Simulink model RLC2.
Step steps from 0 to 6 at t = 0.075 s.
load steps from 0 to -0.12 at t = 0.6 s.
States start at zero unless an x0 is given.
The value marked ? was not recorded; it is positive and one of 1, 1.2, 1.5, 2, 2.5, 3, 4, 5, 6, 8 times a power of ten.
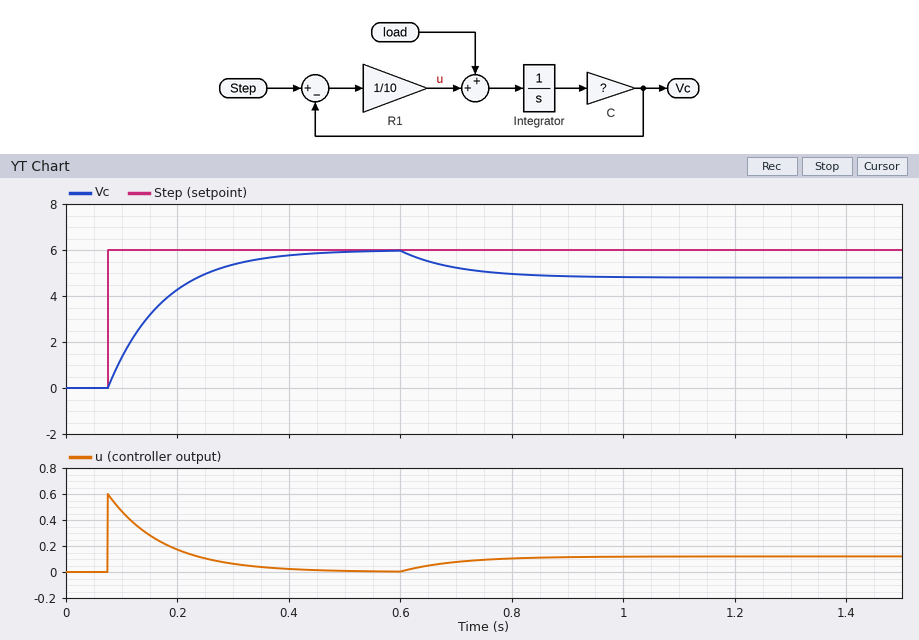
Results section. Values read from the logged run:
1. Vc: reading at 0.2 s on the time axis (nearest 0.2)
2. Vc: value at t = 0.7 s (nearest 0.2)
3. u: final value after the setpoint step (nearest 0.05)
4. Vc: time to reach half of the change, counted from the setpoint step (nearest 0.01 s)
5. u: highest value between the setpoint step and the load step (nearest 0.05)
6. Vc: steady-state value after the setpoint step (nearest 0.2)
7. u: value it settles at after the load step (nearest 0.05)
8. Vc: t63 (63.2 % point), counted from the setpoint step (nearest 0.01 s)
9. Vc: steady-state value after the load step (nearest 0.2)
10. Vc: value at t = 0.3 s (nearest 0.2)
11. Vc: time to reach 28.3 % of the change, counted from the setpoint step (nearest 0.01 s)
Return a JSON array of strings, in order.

["4.2", "5.2", "0.00", "0.07 s", "0.60", "6.0", "0.10", "0.10 s", "4.8", "5.4", "0.03 s"]
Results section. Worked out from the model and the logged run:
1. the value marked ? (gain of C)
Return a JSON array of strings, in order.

["100"]
